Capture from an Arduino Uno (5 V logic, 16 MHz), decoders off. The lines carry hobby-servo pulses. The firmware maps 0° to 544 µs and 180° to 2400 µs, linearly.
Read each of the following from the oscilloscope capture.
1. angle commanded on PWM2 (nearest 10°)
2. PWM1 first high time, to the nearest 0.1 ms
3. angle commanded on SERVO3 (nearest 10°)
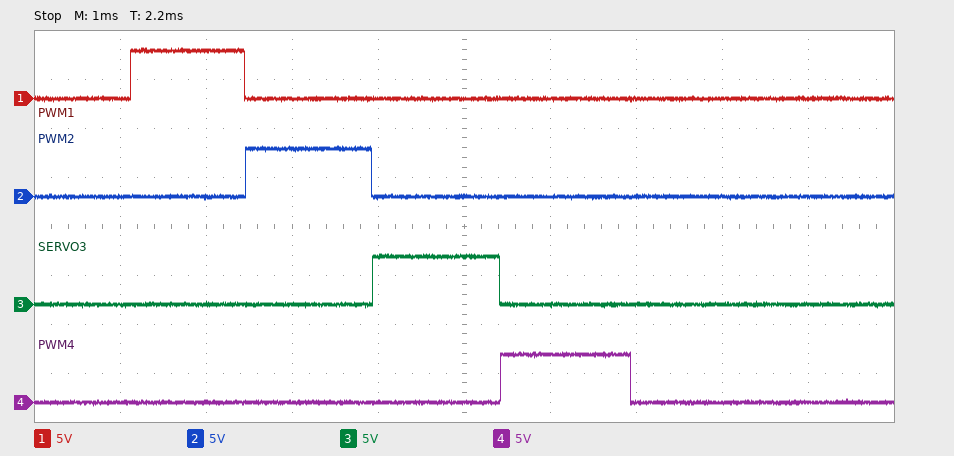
90°
1.3 ms
90°
